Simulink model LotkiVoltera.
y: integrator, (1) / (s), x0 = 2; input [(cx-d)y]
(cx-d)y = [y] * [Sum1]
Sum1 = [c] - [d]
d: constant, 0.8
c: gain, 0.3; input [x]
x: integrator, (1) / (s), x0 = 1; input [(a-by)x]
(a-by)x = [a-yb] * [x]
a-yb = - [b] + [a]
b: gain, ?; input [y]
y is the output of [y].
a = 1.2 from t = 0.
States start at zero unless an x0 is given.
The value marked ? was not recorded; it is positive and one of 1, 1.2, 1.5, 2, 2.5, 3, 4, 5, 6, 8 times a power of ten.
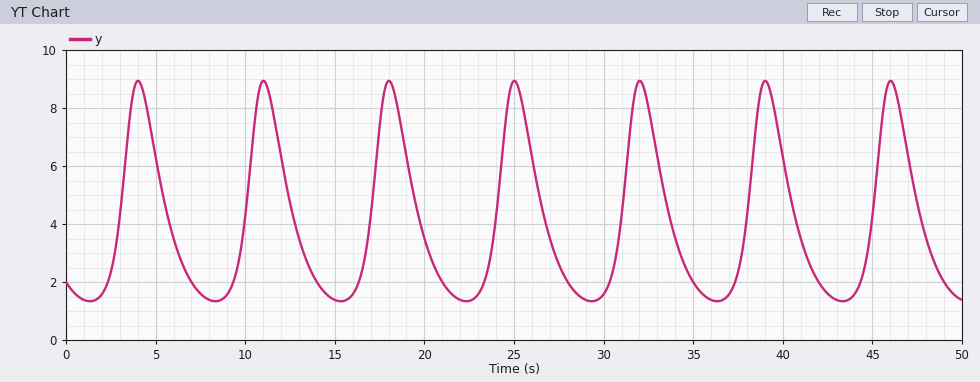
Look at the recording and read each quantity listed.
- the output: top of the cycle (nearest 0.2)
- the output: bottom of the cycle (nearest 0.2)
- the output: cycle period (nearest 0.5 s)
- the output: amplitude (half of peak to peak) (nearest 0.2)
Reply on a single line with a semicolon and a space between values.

9.0; 1.4; 7.0 s; 3.8
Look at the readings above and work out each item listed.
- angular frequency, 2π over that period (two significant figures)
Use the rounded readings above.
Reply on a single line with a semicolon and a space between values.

0.90 rad/s
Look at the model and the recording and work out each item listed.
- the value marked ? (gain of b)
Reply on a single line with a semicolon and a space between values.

0.3
